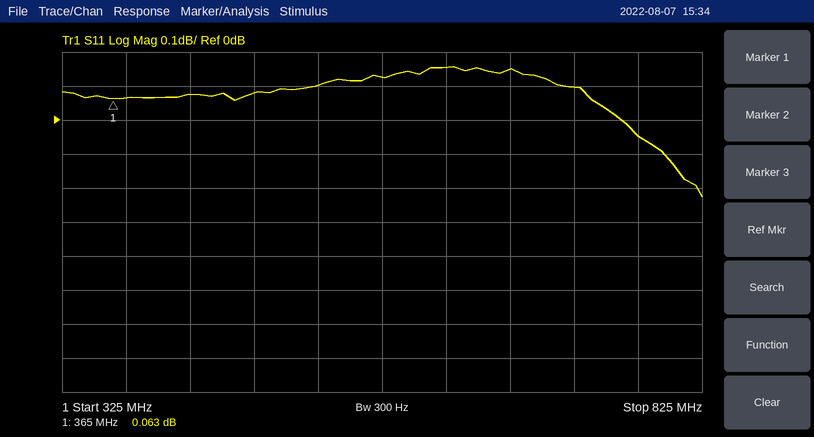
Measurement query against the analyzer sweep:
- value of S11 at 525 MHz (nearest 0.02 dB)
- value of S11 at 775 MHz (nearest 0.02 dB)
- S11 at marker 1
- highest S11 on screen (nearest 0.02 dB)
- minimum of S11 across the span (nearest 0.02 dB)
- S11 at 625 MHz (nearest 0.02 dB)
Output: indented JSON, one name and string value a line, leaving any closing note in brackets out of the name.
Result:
{
  "value of S11 at 525 MHz": "0.10 dB",
  "value of S11 at 775 MHz": "-0.04 dB",
  "S11 at marker 1": "0.063 dB",
  "highest S11 on screen": "0.16 dB",
  "minimum of S11 across the span": "-0.22 dB",
  "S11 at 625 MHz": "0.16 dB"
}
